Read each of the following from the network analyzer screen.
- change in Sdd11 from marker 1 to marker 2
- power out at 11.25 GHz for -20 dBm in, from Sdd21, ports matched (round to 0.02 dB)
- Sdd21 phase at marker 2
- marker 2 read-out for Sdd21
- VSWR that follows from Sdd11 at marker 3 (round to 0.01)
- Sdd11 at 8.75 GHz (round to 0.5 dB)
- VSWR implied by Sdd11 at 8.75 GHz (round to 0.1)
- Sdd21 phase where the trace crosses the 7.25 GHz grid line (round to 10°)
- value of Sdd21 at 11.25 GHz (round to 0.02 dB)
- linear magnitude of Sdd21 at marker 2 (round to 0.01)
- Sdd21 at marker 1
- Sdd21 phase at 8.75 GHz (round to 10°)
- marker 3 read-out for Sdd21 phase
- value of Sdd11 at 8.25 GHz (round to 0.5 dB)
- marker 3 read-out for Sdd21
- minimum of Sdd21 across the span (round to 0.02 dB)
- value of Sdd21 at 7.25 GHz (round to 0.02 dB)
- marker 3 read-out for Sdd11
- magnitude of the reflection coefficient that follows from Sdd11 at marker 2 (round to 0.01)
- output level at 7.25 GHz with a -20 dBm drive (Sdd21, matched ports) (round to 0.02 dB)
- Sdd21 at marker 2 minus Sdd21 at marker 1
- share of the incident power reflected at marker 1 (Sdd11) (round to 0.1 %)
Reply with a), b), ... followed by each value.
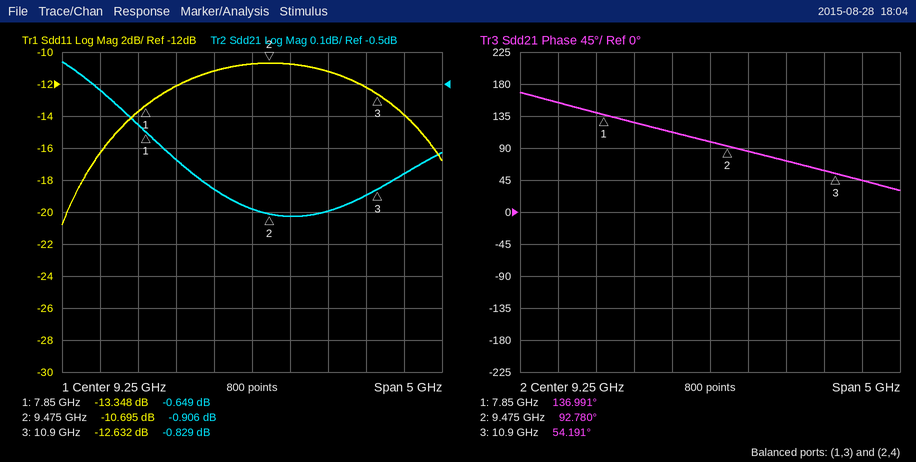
a) 2.653 dB
b) -20.78 dBm
c) 92.780°
d) -0.906 dB
e) 1.61
f) -11.0 dB
g) 1.8
h) 150°
i) -0.78 dB
j) 0.90
k) -0.649 dB
l) 110°
m) 54.191°
n) -12.0 dB
o) -0.829 dB
p) -0.92 dB
q) -0.52 dB
r) -12.632 dB
s) 0.29
t) -20.52 dBm
u) -0.257 dB
v) 4.6 %
